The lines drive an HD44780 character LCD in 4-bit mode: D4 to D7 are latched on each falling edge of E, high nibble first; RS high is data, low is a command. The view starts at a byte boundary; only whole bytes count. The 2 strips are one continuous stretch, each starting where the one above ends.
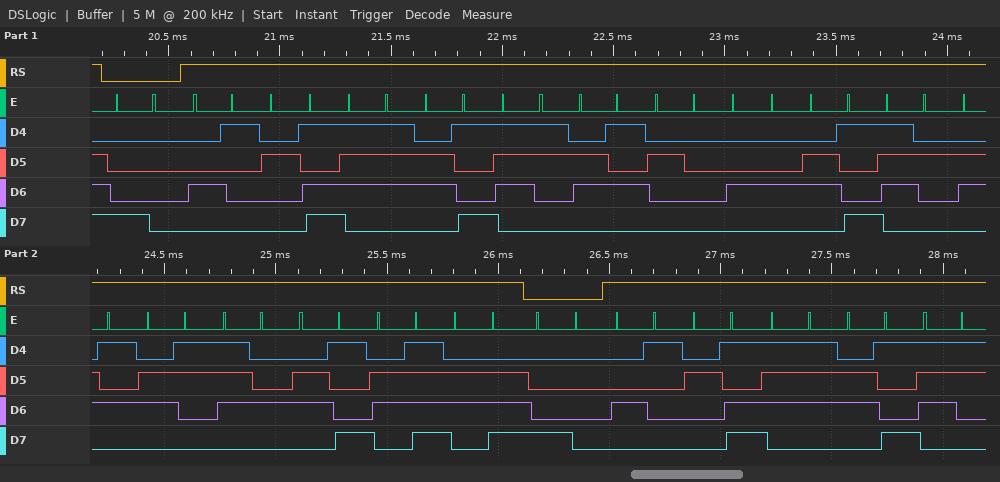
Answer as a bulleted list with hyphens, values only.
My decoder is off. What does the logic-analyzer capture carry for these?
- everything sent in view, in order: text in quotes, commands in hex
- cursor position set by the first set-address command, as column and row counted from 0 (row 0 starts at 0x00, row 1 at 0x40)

- 0x80 "A-wise Direction" 0x80 "A-wis"
- column 0, row 0
